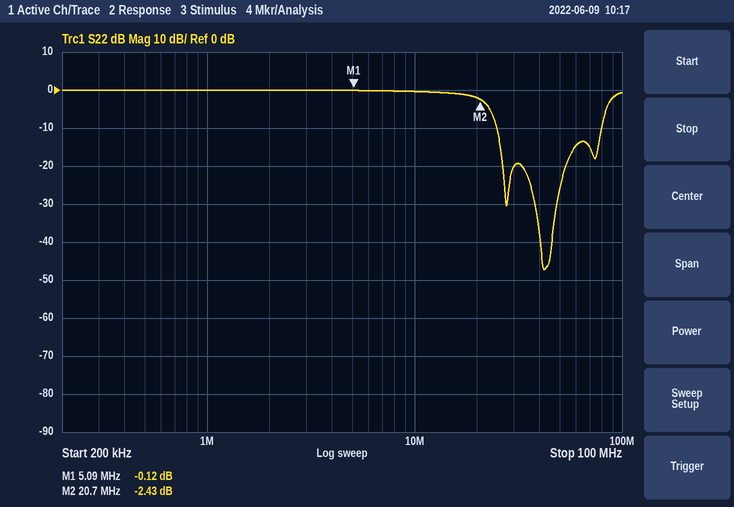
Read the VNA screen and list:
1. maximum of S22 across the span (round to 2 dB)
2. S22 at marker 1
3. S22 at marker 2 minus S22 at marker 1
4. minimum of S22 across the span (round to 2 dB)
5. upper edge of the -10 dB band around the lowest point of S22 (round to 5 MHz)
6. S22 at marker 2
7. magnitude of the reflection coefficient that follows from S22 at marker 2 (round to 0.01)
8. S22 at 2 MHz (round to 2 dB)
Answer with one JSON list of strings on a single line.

["0 dB", "-0.12 dB", "-2.31 dB", "-48 dB", "80 MHz", "-2.43 dB", "0.76", "0 dB"]
